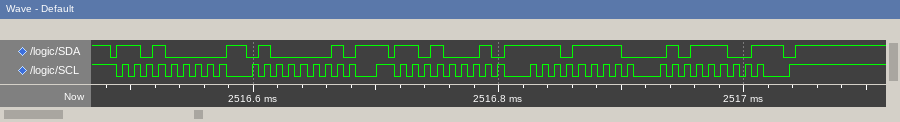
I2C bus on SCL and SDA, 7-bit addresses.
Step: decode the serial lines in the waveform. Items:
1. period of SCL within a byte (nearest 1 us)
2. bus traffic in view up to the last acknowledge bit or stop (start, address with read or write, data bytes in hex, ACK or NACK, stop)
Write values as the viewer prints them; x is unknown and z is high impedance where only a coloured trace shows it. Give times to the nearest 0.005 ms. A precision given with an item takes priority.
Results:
10 us
start, address 68 write ACK, 41 ACK, repeated start, address 68 read ACK, EF ACK, 5C NACK, stop
